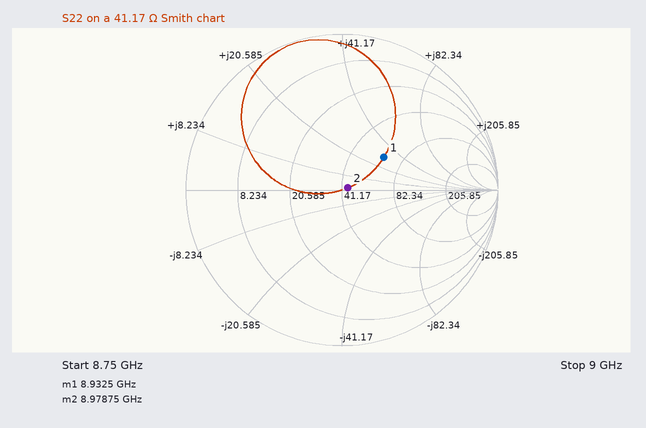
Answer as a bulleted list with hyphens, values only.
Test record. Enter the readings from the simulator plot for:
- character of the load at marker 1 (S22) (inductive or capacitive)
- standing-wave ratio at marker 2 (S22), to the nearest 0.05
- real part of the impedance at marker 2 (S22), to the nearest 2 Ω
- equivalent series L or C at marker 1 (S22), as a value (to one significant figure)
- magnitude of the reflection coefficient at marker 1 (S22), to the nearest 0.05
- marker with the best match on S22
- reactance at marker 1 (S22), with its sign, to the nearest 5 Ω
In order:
- inductive
- 1.10
- 44 Ω
- 500 pH
- 0.35
- marker 2
- +30 Ω
